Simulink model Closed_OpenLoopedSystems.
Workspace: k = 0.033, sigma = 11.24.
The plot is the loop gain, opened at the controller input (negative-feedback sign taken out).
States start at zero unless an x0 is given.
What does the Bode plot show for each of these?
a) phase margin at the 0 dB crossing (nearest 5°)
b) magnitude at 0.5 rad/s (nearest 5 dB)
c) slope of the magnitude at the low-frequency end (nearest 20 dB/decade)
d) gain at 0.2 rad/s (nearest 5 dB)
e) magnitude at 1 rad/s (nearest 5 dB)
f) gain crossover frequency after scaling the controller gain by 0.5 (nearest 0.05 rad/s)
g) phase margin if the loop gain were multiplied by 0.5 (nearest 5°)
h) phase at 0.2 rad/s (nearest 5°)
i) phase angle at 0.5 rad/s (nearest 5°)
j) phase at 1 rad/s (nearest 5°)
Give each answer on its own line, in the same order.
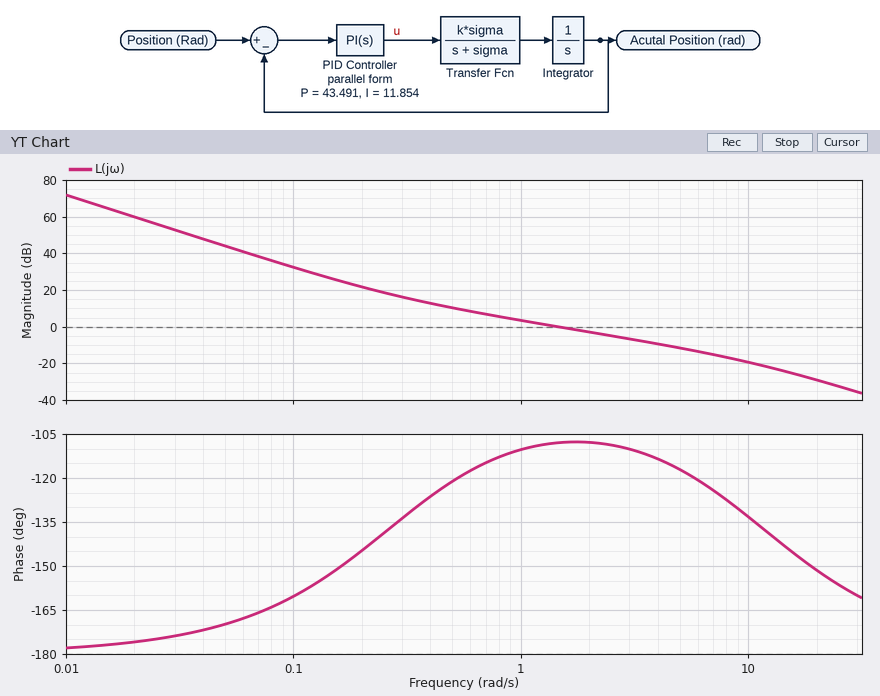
70°
10 dB
-40 dB/decade
20 dB
5 dB
0.75 rad/s
65°
-145°
-120°
-110°
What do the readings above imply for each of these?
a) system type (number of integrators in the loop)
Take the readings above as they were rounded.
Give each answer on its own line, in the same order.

2
